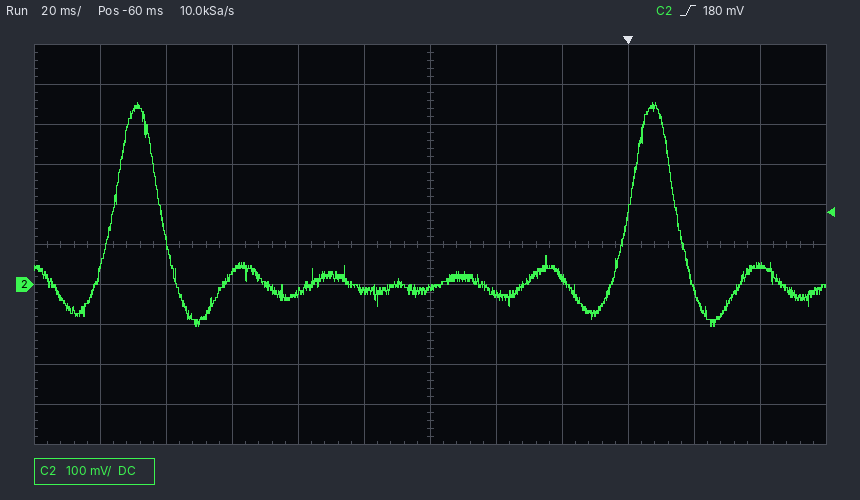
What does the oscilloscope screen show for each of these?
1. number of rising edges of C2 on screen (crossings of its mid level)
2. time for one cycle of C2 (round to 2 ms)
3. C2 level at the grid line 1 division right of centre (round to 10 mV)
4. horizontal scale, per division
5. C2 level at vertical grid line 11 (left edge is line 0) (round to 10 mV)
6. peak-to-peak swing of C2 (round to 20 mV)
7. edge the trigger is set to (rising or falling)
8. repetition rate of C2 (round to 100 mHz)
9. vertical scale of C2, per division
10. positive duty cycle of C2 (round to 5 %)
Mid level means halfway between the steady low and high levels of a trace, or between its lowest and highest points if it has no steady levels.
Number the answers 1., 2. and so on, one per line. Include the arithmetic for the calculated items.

1. 2
2. 156 ms
3. -20 mV
4. 20 ms
5. 50 mV
6. 560 mV
7. rising
8. 1 / 156 ms ≈ 6.4 Hz
9. 100 mV
10. 10 %
